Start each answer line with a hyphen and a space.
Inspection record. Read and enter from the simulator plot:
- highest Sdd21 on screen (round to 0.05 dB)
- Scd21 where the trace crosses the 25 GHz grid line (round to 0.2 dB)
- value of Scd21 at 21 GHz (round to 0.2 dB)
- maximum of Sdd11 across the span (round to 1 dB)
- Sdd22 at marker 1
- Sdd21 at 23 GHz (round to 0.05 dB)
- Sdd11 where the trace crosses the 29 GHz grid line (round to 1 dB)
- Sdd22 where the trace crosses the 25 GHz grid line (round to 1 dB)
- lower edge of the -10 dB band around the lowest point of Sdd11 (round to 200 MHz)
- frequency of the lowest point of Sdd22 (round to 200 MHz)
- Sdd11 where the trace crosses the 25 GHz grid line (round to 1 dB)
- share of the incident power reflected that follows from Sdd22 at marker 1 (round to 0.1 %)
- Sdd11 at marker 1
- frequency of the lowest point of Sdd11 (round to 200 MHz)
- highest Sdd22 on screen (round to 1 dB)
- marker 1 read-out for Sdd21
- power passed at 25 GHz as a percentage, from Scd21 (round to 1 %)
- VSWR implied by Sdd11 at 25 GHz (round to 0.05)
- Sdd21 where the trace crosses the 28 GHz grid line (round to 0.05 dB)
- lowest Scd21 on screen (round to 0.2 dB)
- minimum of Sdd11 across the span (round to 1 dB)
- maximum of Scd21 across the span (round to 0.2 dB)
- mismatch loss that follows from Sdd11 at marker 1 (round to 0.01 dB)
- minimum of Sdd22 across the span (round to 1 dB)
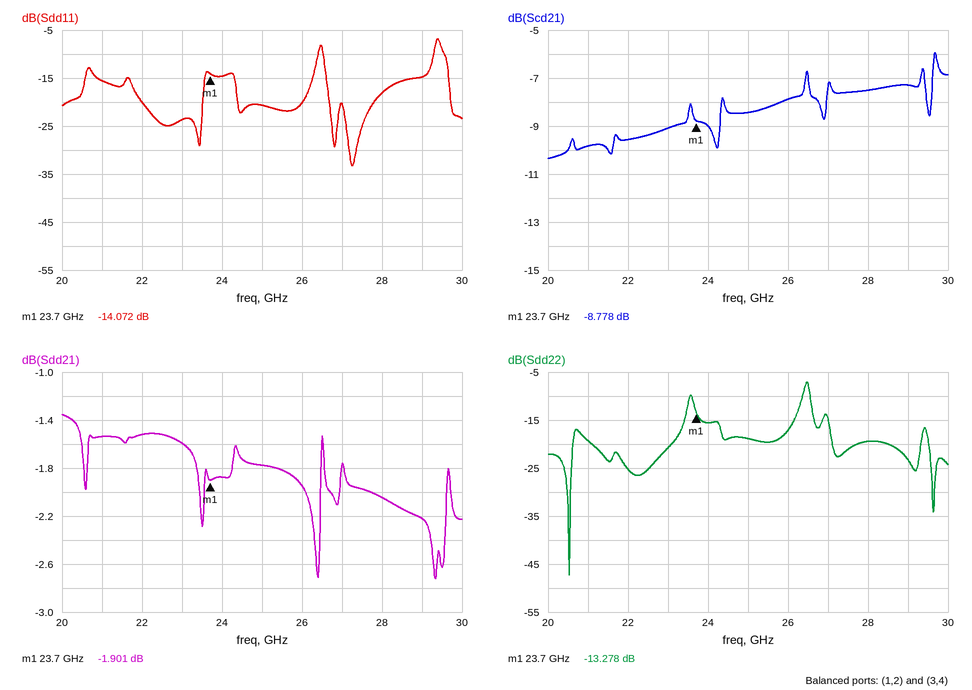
- -1.35 dB
- -8.4 dB
- -9.8 dB
- -7 dB
- -13.278 dB
- -1.60 dB
- -15 dB
- -19 dB
- 26.6 GHz
- 20.6 GHz
- -21 dB
- 4.7 %
- -14.072 dB
- 27.2 GHz
- -7 dB
- -1.901 dB
- 14 %
- 1.20
- -2.05 dB
- -10.4 dB
- -33 dB
- -6.0 dB
- 0.17 dB
- -47 dB
